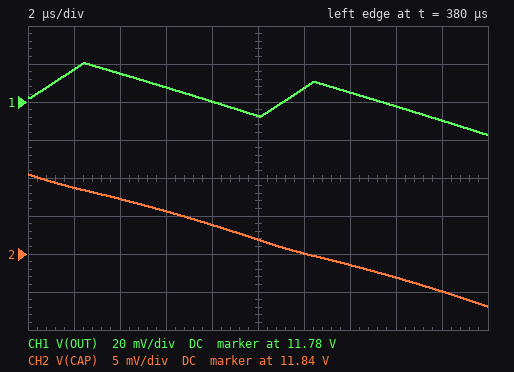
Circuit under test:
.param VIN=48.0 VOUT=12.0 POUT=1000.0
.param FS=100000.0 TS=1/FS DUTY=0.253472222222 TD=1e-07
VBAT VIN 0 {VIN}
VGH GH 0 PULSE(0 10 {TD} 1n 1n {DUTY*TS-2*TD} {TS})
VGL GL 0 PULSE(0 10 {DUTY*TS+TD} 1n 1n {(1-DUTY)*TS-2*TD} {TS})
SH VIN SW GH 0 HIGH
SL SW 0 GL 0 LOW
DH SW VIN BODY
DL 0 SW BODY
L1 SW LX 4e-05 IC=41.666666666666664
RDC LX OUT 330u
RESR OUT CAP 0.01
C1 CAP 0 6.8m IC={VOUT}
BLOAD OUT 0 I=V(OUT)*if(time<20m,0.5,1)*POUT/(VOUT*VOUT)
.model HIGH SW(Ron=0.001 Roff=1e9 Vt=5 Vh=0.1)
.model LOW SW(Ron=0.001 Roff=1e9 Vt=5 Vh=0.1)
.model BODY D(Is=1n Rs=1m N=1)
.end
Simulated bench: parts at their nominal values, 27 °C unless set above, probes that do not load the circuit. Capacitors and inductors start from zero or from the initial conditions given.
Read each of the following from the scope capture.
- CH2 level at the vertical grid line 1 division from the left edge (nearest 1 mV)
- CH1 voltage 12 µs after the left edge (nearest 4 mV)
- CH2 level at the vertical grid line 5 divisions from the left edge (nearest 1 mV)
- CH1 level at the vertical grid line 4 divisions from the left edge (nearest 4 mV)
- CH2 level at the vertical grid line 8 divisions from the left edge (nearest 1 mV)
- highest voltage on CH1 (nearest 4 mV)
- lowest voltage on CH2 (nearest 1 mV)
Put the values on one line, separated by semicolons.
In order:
11.849 V; 11.788 V; 11.842 V; 11.780 V; 11.837 V; 11.800 V; 11.833 V
